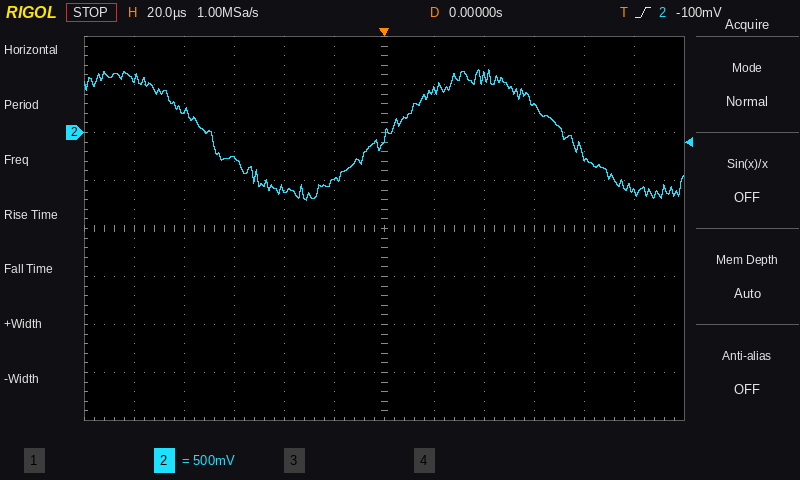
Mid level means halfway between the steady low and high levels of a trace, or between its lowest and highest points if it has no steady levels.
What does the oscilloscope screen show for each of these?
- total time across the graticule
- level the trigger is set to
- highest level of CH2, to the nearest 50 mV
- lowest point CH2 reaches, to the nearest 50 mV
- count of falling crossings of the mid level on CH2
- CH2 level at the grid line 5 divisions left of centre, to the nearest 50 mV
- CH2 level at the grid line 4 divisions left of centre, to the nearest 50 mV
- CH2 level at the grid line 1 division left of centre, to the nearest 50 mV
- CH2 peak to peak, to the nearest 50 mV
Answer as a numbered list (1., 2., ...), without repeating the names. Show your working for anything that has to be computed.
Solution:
1. 240 µs
2. -100 mV
3. 650 mV
4. -700 mV
5. 2
6. 550 mV
7. 250 mV
8. -500 mV
9. 650 mV − (-700 mV) = 1.35 V
